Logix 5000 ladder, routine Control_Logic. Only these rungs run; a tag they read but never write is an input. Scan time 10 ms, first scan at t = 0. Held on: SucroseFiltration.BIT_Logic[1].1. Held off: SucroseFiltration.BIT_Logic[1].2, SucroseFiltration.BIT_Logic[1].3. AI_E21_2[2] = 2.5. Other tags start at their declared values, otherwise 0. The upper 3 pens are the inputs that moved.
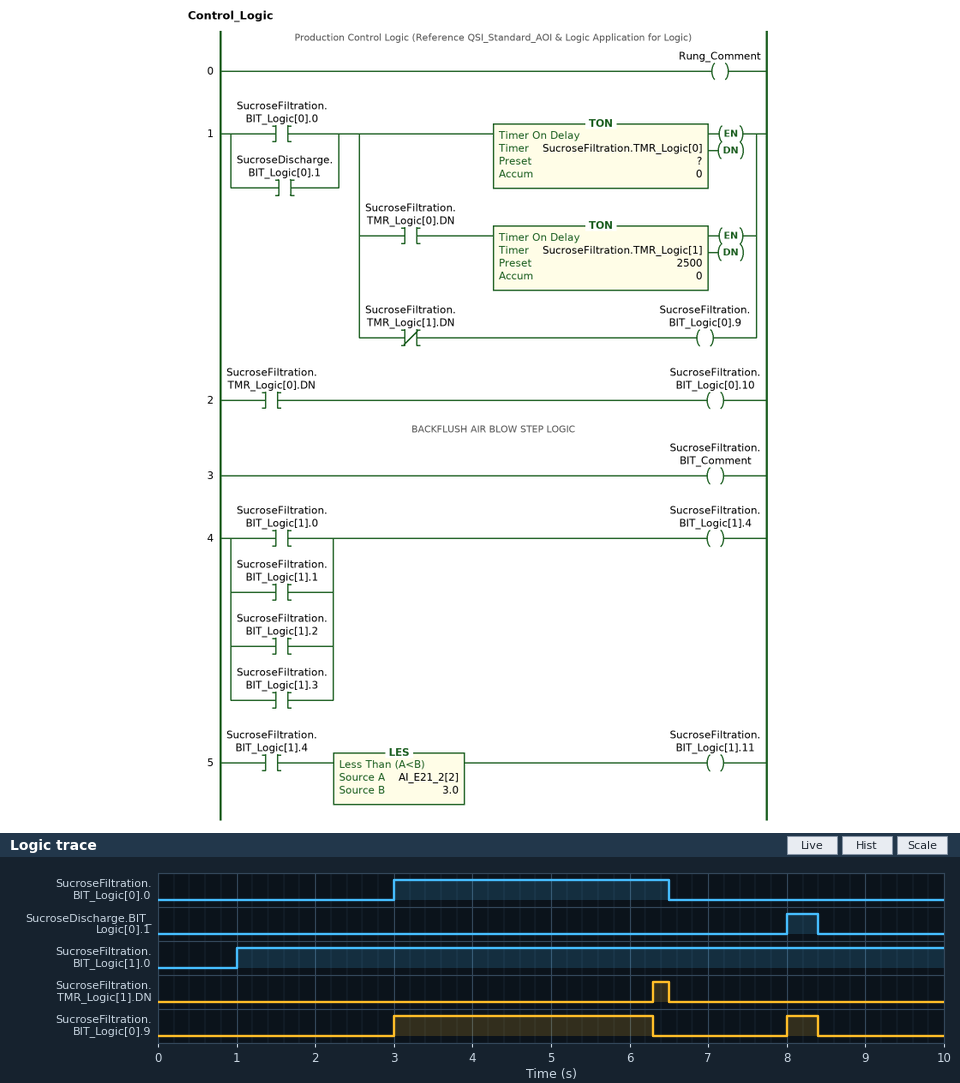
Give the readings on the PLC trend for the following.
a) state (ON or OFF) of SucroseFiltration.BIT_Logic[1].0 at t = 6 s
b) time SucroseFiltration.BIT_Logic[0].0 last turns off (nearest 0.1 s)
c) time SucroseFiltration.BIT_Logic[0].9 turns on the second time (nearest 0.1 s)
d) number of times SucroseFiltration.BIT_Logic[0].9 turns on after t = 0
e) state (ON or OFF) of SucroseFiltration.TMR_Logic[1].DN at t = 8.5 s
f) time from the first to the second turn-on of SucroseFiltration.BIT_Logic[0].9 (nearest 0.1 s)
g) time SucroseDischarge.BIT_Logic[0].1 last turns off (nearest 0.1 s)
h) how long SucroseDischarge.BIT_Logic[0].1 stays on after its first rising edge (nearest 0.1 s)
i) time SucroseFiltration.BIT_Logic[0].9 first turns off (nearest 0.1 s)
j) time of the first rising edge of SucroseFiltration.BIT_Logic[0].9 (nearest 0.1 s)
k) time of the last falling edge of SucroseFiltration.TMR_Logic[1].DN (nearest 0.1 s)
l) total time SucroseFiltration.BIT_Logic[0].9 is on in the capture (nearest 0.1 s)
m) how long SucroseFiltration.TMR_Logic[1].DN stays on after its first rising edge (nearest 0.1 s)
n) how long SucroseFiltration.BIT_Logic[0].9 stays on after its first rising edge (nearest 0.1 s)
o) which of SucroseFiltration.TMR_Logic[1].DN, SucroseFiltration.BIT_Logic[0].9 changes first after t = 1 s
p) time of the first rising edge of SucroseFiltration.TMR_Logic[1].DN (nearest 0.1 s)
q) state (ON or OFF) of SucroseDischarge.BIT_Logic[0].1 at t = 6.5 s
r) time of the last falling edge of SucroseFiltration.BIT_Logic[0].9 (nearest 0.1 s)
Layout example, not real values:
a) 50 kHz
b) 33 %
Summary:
a) ON
b) 6.5 s
c) 8.0 s
d) 2
e) OFF
f) 5.0 s
g) 8.4 s
h) 0.4 s
i) 6.3 s
j) 3.0 s
k) 6.5 s
l) 3.7 s
m) 0.2 s
n) 3.3 s
o) SucroseFiltration.BIT_Logic[0].9
p) 6.3 s
q) OFF
r) 8.4 s
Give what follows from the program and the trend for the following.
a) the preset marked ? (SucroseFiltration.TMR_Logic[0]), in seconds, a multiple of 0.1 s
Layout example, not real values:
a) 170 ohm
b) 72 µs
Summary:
a) 0.8 s
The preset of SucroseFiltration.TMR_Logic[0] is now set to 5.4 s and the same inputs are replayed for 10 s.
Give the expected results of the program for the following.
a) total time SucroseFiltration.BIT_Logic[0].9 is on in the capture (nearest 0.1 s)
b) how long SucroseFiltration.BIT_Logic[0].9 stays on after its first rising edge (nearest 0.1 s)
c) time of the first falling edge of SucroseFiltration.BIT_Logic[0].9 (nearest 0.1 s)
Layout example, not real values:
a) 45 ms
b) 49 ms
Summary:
a) 3.9 s
b) 3.5 s
c) 6.5 s
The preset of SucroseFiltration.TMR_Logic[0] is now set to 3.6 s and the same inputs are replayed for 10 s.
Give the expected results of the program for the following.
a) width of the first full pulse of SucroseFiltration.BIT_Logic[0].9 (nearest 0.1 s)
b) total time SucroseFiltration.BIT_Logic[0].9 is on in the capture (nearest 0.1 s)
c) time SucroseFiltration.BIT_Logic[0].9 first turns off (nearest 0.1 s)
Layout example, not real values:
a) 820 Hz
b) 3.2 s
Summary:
a) 3.5 s
b) 3.9 s
c) 6.5 s
